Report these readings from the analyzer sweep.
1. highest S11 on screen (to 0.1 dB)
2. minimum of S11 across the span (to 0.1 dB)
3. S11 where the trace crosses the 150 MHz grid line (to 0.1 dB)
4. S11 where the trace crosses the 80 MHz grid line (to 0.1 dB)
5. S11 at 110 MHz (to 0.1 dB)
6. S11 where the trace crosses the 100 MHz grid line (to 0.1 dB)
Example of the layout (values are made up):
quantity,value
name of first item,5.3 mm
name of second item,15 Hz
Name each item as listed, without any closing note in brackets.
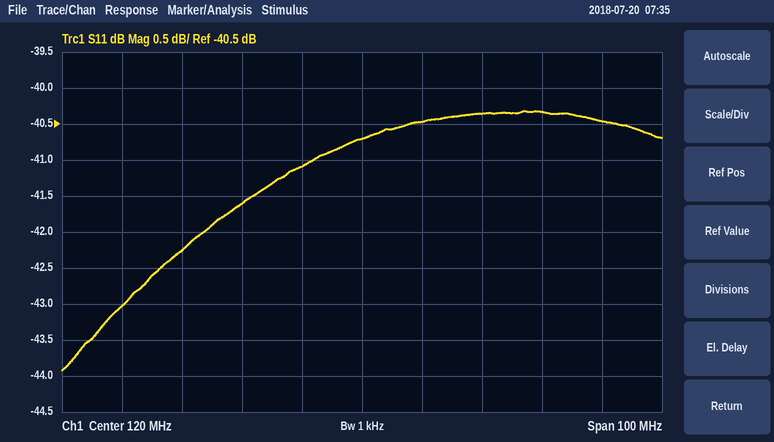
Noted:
quantity,value
highest S11 on screen,-40.3 dB
minimum of S11 across the span,-43.9 dB
S11 where the trace crosses the 150 MHz grid line,-40.3 dB
S11 where the trace crosses the 80 MHz grid line,-43.0 dB
S11 at 110 MHz,-41.1 dB
S11 where the trace crosses the 100 MHz grid line,-41.6 dB
